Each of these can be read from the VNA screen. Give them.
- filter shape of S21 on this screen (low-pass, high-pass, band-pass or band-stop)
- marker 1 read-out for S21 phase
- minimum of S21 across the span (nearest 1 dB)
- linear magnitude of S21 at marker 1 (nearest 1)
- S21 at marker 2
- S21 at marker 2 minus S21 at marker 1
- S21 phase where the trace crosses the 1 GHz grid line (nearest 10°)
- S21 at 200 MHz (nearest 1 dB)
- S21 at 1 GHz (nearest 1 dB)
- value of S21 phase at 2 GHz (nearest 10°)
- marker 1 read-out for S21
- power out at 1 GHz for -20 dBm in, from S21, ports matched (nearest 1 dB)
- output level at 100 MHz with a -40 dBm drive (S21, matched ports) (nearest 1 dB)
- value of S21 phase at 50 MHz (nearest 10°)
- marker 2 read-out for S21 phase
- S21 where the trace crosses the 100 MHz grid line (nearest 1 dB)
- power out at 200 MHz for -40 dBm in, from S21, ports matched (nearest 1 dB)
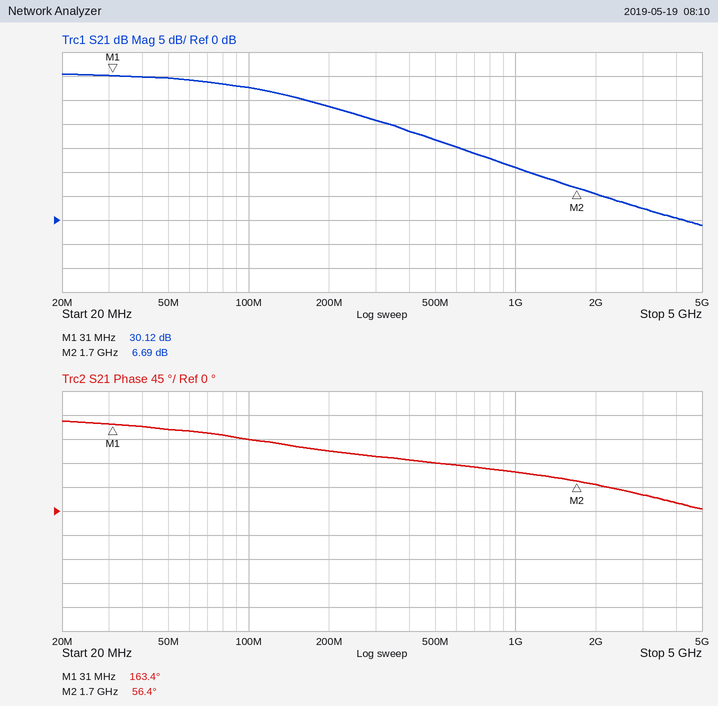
low-pass
163.4°
-1 dB
32
6.69 dB
-23.43 dB
70°
24 dB
11 dB
50°
30.12 dB
-9 dBm
-12 dBm
150°
56.4°
28 dB
-16 dBm
